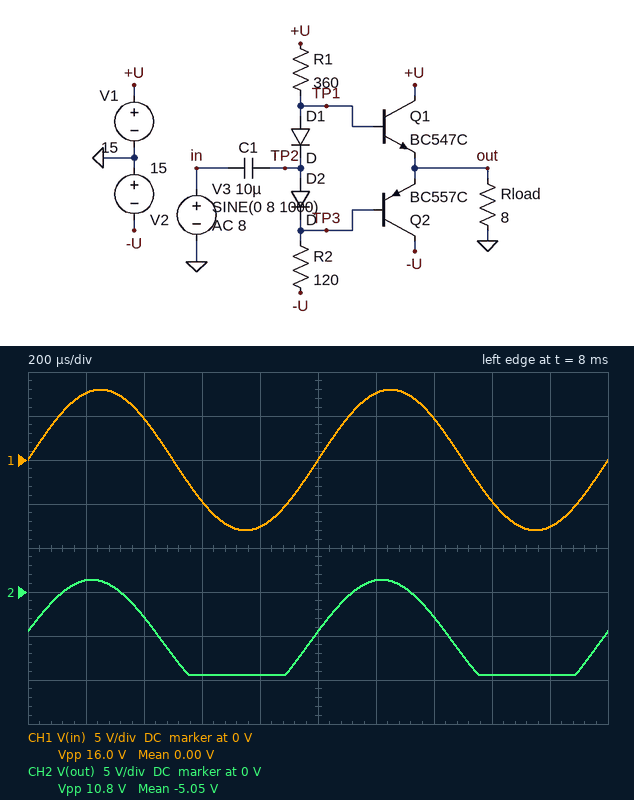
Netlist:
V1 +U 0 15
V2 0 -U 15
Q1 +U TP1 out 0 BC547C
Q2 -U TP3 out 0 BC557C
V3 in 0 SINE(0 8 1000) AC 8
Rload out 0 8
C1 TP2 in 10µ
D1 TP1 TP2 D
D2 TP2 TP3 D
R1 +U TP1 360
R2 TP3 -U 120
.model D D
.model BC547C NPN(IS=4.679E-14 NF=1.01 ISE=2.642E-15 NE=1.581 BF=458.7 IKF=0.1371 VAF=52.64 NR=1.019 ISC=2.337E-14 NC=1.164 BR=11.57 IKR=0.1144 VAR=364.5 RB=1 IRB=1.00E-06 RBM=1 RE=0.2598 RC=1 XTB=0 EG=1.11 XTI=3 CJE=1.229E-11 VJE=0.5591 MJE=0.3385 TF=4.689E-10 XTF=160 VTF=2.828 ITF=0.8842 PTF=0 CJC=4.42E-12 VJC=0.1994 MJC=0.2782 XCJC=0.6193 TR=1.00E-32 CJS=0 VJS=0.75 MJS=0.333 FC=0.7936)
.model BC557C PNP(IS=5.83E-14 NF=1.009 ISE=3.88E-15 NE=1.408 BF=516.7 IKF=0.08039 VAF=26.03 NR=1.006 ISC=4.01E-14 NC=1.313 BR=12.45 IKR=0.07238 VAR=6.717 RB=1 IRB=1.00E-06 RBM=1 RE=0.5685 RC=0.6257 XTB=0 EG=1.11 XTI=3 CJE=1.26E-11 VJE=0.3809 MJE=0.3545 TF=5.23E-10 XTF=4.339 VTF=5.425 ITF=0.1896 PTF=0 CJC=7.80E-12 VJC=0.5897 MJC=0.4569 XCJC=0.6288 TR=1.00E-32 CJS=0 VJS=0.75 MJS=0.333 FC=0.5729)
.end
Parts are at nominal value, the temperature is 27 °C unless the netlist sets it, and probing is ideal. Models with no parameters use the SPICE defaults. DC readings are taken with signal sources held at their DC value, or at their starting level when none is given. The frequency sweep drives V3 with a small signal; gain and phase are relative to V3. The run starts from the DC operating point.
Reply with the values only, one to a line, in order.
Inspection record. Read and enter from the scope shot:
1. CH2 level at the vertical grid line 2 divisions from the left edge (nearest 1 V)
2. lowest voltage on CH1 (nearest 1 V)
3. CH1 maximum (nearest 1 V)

-3 V
-8 V
8 V
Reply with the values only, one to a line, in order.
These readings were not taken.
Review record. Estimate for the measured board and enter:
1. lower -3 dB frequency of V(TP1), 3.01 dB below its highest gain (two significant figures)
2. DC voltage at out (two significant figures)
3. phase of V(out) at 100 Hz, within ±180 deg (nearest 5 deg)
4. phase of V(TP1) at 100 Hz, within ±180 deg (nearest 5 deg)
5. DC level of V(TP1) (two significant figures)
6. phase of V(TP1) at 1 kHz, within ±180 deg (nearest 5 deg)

230 Hz
-5.7 V
65 deg
65 deg
-5.5 V
15 deg
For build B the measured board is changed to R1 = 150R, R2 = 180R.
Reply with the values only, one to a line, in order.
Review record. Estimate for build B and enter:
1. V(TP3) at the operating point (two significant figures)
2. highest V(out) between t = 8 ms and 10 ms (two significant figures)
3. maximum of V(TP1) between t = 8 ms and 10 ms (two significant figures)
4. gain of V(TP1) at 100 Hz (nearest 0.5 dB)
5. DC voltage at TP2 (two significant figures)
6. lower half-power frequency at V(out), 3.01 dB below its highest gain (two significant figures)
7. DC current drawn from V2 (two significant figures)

470 mV
8.5 V
9.7 V
-7.0 dB
1.2 V
200 Hz
120 mA
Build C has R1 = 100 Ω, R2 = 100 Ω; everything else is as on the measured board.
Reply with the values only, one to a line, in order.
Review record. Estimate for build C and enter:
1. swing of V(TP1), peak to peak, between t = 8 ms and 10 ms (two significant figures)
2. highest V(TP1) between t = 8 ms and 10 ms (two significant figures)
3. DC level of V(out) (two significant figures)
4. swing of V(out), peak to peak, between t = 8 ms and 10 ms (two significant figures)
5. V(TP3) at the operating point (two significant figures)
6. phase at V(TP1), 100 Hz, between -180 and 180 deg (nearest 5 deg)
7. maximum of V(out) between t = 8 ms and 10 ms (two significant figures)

15 V
8.4 V
11 mV
14 V
-780 mV
75 deg
7.3 V
